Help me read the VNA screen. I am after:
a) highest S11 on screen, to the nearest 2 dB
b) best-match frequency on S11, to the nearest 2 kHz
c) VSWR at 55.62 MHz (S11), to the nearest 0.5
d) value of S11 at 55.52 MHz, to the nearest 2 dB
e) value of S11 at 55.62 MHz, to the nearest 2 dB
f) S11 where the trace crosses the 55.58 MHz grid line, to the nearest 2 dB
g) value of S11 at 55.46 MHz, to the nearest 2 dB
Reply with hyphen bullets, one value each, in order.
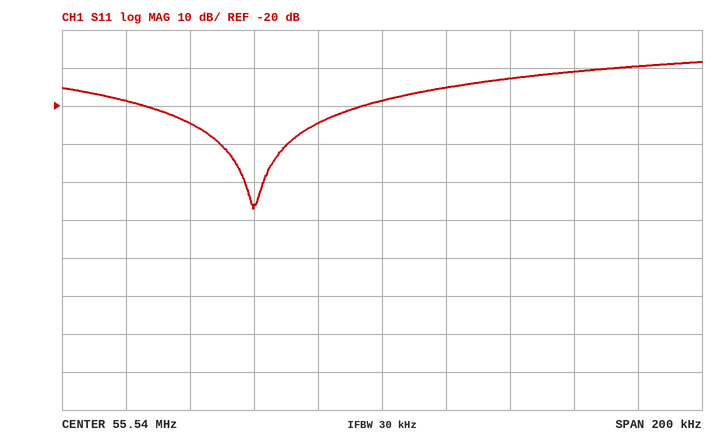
- -8 dB
- 55.500 MHz
- 2.0
- -24 dB
- -10 dB
- -12 dB
- -18 dB
